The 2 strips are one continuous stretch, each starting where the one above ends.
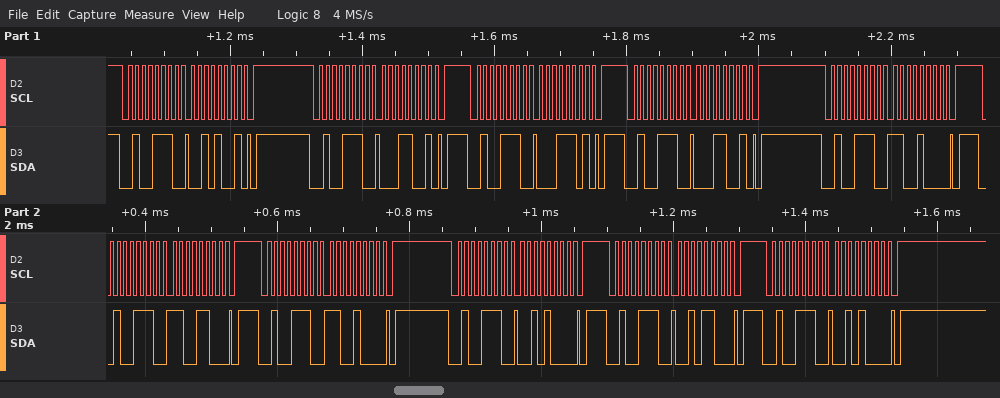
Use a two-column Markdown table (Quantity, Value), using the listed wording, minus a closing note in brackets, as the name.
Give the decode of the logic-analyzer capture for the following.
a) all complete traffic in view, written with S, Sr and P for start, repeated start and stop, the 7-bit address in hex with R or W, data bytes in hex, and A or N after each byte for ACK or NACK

| Quantity | Value |
|---|---|
| all complete traffic in view, written with S, Sr and P for start, repeated start and stop, the 7-bit address in hex with R or W, data bytes in hex, and A or N after each byte for ACK or NACK | S 27W A 29 A P S 27W A 19 A P S 27W A 1D A P S 27W A 19 A P S 27W A C8 A P S 27W A CC A P S 27W A C8 A P S 27W A 28 A P S 27W A 2C A P S 27W A 28 A P |
